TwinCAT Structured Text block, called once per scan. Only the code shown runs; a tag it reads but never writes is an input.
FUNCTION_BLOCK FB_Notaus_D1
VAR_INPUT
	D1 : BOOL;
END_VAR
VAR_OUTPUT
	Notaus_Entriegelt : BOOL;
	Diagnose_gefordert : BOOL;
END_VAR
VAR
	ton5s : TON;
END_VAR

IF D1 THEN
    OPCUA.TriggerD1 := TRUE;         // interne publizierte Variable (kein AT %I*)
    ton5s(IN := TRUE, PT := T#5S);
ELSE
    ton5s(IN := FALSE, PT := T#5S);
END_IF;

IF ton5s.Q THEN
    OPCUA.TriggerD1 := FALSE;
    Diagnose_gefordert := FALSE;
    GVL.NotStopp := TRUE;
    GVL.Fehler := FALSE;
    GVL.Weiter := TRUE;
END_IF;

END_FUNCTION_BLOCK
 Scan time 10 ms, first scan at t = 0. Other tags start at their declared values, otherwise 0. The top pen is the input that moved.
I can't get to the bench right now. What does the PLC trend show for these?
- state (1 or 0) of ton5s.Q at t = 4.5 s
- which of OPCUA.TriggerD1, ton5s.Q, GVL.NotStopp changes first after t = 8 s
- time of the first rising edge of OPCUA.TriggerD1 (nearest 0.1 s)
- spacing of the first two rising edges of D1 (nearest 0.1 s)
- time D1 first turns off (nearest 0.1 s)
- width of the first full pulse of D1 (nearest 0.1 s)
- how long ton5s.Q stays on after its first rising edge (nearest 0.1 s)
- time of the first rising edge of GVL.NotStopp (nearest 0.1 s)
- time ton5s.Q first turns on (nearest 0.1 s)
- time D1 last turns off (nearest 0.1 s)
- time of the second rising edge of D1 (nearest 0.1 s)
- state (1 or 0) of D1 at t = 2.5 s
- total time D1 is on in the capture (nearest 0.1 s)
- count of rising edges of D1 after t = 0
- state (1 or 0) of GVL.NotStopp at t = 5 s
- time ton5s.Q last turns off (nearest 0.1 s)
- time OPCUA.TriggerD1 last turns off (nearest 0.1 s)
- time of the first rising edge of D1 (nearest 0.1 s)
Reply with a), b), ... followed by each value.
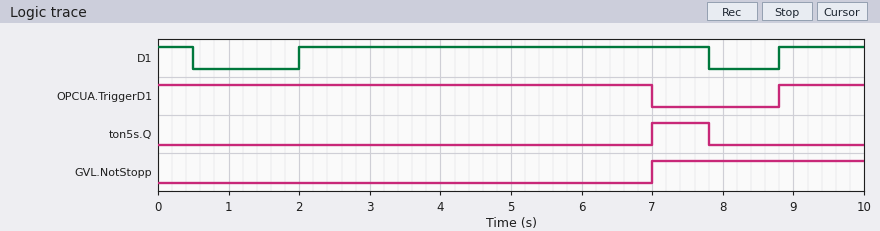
a) 0
b) OPCUA.TriggerD1
c) 8.8 s
d) 6.8 s
e) 0.5 s
f) 5.8 s
g) 0.8 s
h) 7.0 s
i) 7.0 s
j) 7.8 s
k) 8.8 s
l) 1
m) 7.5 s
n) 2
o) 0
p) 7.8 s
q) 7.0 s
r) 2.0 s
